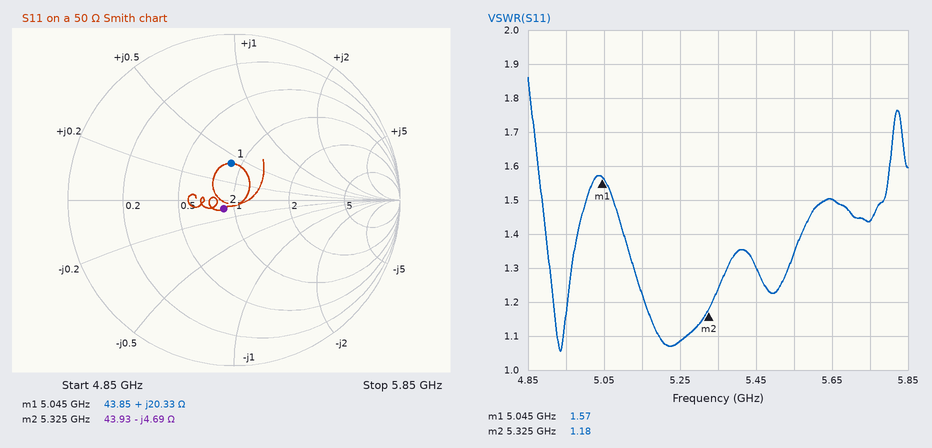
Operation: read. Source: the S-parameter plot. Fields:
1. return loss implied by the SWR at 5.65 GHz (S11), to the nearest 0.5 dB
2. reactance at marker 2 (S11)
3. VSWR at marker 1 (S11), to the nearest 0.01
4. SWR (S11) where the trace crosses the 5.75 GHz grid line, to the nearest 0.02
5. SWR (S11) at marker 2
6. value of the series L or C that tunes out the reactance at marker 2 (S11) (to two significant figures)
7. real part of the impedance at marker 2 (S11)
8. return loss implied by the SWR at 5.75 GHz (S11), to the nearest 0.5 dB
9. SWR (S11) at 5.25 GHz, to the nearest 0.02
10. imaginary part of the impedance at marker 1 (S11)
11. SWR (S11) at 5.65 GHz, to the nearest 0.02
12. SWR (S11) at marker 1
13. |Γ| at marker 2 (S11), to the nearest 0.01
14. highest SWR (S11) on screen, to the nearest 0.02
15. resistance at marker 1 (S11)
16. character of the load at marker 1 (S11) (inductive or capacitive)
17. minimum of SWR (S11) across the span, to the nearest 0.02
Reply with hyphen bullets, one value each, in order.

- 14.0 dB
- -4.69 Ω
- 1.57
- 1.44
- 1.18
- 140 pH
- 43.93 Ω
- 15.0 dB
- 1.08
- +20.33 Ω
- 1.50
- 1.57
- 0.08
- 1.86
- 43.85 Ω
- inductive
- 1.06
